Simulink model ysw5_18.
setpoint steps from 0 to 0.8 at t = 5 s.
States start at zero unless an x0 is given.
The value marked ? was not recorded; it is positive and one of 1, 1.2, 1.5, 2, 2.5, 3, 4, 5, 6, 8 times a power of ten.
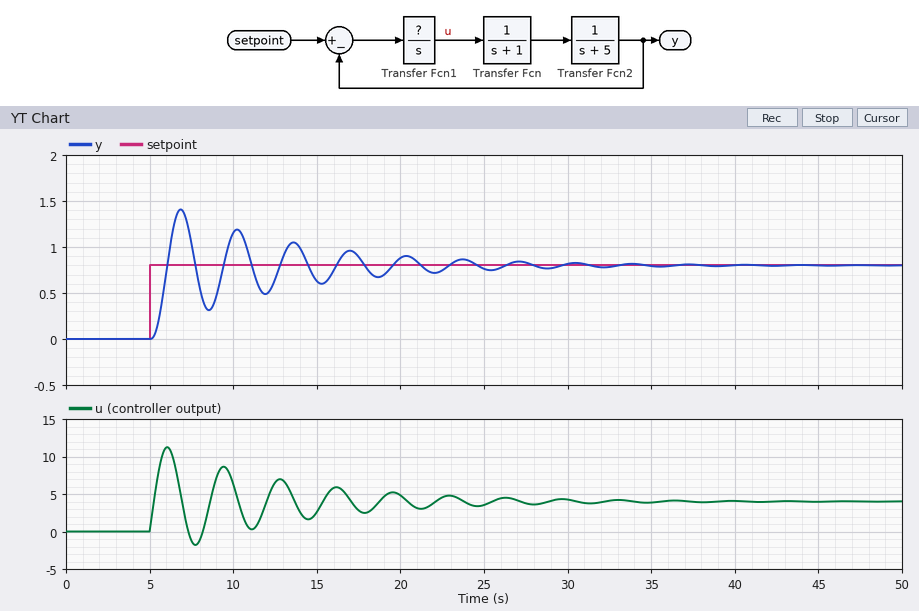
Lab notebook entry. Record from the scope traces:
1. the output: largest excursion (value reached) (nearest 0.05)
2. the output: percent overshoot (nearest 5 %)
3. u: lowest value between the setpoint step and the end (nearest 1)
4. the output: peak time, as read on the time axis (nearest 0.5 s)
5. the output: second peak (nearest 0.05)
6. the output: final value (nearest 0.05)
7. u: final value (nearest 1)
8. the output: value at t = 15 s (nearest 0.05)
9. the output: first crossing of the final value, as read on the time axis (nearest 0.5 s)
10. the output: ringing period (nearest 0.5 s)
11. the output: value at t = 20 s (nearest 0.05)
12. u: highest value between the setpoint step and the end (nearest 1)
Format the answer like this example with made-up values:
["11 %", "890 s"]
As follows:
["1.40", "75 %", "-2", "7.0 s", "1.20", "0.80", "4", "0.65", "6.0 s", "3.5 s", "0.90", "11"]
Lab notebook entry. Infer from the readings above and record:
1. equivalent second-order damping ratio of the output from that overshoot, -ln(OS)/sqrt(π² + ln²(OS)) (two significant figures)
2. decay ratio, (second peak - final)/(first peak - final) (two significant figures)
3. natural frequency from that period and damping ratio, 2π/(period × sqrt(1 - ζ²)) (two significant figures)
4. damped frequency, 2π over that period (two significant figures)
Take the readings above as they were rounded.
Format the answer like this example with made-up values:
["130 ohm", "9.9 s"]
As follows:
["0.091", "0.67", "1.8 rad/s", "1.8 rad/s"]
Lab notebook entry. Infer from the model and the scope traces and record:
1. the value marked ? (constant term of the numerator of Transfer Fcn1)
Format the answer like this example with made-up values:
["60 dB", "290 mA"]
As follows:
["20"]
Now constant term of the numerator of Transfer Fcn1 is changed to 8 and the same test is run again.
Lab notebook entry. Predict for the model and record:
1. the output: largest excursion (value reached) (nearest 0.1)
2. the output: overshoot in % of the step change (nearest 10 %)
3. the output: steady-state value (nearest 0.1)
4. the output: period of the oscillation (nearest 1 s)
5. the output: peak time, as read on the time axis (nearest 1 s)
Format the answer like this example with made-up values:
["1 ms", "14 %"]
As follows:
["1.1", "40 %", "0.8", "5 s", "8 s"]
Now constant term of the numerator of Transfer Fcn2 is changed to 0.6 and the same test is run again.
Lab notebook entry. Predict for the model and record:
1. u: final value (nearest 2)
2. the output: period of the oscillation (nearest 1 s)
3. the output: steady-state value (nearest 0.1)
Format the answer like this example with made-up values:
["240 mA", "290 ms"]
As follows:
["6", "4 s", "0.8"]
